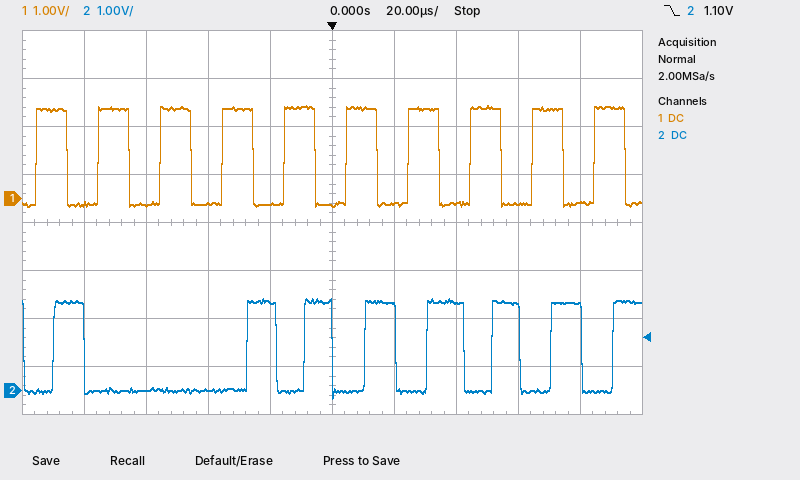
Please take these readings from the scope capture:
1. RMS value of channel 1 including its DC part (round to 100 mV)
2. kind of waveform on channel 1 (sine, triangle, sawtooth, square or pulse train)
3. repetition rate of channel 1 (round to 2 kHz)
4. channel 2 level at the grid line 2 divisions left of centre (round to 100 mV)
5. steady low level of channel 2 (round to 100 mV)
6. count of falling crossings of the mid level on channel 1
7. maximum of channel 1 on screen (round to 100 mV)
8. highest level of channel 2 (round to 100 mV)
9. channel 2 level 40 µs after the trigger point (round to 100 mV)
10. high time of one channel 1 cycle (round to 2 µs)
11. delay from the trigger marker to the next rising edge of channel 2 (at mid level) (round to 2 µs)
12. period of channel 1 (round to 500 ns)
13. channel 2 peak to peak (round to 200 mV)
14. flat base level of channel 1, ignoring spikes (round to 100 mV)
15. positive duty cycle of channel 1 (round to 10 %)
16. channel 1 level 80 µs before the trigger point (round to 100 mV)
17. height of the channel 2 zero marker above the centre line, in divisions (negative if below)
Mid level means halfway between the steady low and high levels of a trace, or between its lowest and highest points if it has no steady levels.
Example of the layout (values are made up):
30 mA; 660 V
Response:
1.3 V; square; 50 kHz; 0.0 V; 0.0 V; 10; 1.9 V; 1.9 V; 1.8 V; 10 µs; 10 µs; 20.0 µs; 2.0 V; -100 mV; 50 %; -100 mV; -3.5 div
